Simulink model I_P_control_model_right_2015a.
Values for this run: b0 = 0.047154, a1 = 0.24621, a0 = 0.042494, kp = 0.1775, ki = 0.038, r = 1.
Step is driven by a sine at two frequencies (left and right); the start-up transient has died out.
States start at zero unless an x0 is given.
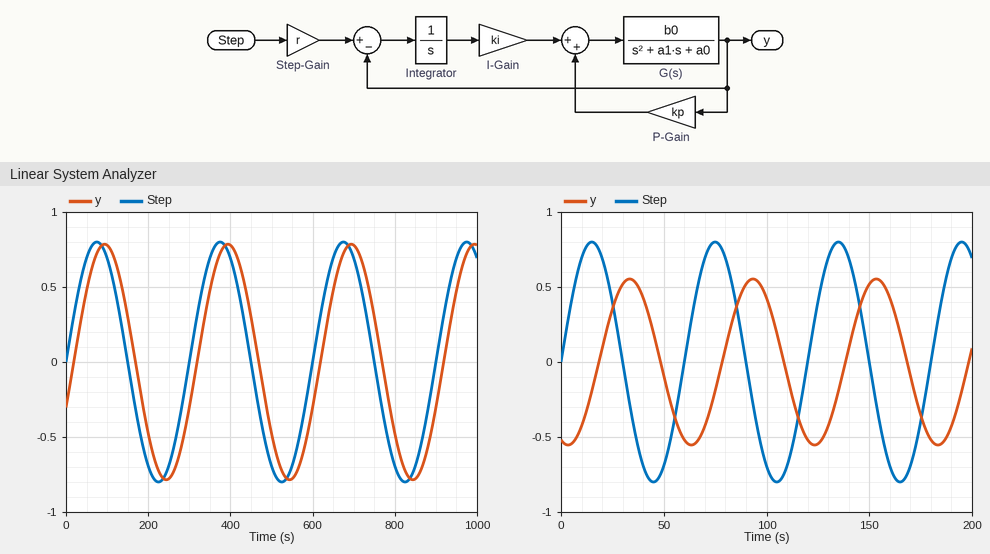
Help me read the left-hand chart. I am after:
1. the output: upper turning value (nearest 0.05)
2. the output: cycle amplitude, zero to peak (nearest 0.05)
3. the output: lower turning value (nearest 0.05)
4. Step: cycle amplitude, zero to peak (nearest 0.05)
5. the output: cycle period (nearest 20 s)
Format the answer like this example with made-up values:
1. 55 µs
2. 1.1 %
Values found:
1. 0.80
2. 0.80
3. -0.80
4. 0.80
5. 300 s
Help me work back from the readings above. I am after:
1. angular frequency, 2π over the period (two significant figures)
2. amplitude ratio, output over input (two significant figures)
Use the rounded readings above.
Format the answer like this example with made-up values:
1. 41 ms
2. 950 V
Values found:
1. 0.021 rad/s
2. 1.0
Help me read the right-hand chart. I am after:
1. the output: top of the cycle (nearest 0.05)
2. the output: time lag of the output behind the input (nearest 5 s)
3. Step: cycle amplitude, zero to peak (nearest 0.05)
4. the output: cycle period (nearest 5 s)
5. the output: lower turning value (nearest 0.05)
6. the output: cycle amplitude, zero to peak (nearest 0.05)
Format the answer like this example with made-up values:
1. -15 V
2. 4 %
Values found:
1. 0.55
2. 20 s
3. 0.80
4. 60 s
5. -0.55
6. 0.55
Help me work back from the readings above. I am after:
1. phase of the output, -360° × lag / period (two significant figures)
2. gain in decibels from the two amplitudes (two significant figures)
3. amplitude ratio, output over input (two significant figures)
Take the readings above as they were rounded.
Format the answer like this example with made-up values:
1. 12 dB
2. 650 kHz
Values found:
1. -120°
2. -3.3 dB
3. 0.69
